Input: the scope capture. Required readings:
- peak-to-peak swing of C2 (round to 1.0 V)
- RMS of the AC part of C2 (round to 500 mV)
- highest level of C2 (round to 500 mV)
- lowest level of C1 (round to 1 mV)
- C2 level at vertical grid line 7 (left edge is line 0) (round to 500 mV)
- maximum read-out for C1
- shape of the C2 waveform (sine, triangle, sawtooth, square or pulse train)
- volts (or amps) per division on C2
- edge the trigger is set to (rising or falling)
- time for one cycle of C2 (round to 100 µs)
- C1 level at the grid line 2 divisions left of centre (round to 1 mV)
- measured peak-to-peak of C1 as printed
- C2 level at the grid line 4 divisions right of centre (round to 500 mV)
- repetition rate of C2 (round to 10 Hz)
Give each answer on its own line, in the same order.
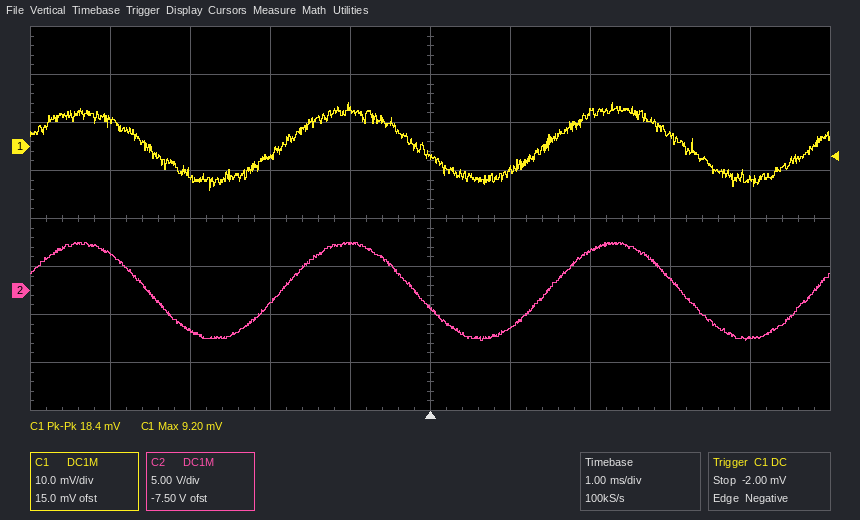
10.0 V
3.5 V
5.0 V
-9 mV
4.0 V
9.20 mV
sine
5 V
falling
3.3 ms
-2 mV
18.4 mV
-5.0 V
300 Hz
